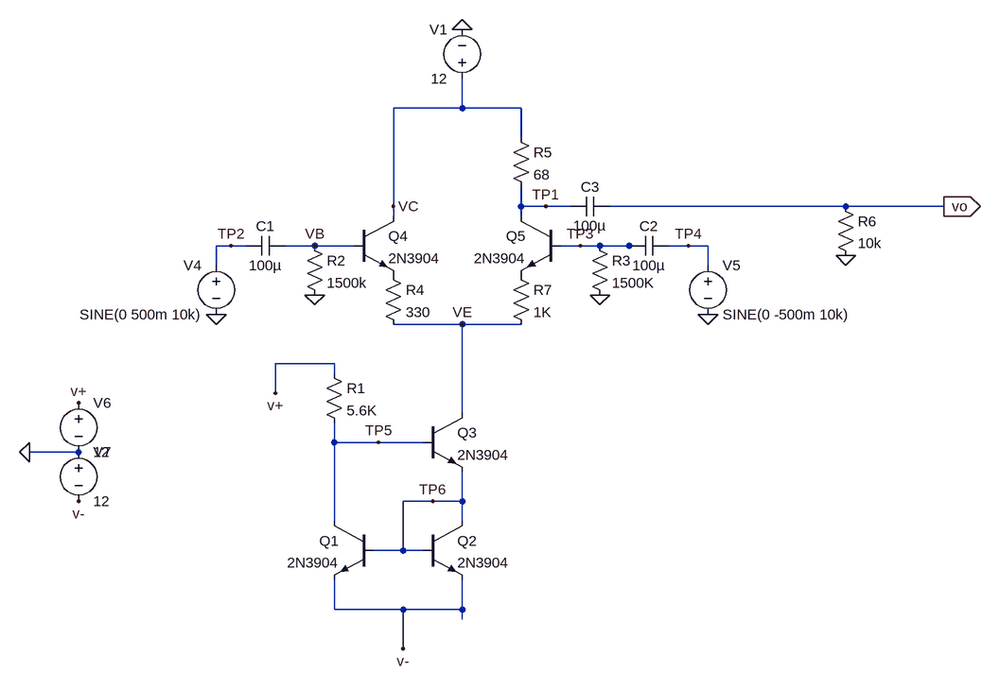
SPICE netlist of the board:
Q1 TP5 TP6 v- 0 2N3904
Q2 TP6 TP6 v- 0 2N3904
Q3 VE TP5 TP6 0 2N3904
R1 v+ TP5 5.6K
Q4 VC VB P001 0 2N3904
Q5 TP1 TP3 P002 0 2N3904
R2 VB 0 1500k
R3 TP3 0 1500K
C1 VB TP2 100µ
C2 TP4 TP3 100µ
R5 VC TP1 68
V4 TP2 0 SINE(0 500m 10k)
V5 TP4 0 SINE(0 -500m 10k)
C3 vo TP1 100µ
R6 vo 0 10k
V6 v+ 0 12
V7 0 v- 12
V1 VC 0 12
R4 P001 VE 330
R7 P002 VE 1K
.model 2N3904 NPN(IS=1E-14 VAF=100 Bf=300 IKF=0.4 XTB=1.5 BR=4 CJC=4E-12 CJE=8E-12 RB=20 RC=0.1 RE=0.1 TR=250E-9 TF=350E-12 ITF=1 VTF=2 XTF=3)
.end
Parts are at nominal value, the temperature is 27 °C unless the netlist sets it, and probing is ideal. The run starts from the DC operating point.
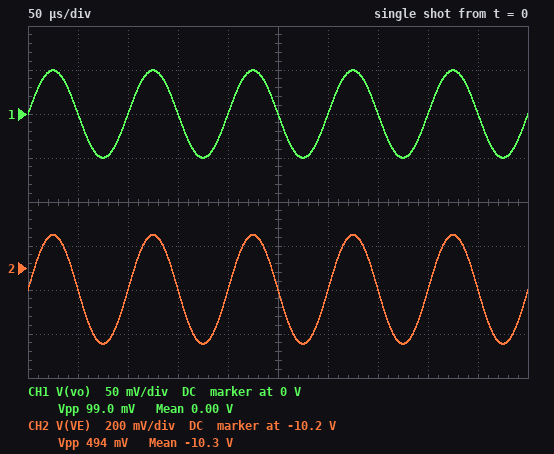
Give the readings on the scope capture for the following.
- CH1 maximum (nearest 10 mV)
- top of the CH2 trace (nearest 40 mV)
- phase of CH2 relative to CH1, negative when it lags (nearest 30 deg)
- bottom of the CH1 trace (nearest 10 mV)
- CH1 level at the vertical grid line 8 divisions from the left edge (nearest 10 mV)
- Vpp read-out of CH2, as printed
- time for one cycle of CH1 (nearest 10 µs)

50 mV
-10.04 V
0 deg
-50 mV
0 V
494 mV
100 µs
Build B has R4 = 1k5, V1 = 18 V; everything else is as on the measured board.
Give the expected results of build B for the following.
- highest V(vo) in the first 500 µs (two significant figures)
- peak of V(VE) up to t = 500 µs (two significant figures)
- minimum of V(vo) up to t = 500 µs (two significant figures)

28 mV
-11 V
-27 mV
